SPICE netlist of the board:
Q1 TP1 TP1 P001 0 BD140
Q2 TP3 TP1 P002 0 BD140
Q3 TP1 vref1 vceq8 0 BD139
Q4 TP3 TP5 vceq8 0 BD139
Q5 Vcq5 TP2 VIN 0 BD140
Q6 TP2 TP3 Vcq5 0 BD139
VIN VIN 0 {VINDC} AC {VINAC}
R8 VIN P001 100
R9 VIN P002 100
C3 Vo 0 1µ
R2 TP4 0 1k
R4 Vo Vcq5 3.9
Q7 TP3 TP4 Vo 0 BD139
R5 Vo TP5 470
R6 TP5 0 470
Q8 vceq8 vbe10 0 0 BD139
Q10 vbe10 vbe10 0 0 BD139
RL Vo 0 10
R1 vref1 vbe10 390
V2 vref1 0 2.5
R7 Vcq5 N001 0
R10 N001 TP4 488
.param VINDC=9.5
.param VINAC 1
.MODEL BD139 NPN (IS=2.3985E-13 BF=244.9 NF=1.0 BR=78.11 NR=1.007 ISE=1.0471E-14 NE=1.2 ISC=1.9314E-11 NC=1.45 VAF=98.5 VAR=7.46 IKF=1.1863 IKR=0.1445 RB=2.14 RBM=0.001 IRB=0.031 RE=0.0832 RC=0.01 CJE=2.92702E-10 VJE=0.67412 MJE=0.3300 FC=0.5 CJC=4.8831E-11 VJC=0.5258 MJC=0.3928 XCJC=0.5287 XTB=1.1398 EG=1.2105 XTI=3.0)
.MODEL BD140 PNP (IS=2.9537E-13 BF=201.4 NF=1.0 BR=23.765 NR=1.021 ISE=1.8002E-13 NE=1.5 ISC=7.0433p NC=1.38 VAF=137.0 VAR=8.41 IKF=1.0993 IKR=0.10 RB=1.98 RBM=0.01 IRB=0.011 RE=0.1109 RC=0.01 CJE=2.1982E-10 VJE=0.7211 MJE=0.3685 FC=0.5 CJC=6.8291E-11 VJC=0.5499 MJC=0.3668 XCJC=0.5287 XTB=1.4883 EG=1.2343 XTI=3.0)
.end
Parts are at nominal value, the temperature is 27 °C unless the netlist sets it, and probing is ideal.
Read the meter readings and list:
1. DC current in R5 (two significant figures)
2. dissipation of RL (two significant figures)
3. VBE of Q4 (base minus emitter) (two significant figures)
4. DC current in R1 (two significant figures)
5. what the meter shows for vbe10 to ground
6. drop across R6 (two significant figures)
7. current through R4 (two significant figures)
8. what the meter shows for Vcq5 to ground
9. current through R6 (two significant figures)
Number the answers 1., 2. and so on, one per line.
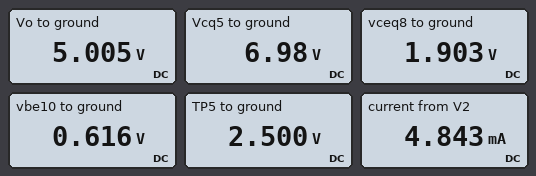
1. 5.3 mA
2. 2.5 W
3. 600 mV
4. 4.8 mA
5. 0.616 V
6. 2.5 V
7. 510 mA
8. 6.98 V
9. 5.3 mA
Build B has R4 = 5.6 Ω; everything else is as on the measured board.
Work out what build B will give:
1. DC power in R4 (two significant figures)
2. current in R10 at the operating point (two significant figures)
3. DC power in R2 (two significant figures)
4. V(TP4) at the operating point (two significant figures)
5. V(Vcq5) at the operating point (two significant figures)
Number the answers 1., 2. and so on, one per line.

1. 1.4 W
2. 5.3 mA
3. 28 mW
4. 5.3 V
5. 7.8 V
